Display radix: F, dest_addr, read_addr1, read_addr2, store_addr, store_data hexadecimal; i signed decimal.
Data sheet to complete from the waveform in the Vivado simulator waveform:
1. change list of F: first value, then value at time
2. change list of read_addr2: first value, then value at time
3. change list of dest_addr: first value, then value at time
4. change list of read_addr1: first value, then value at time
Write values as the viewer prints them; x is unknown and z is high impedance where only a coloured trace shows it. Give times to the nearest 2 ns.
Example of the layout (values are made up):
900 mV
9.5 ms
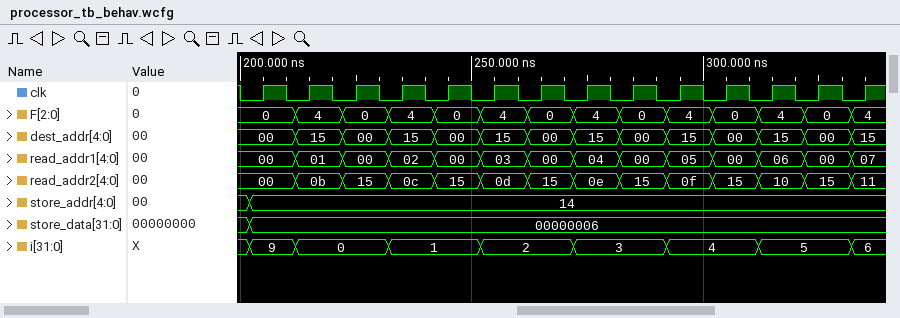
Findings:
0, 4 at 212 ns, 0 at 222 ns, 4 at 232 ns, 0 at 242 ns, 4 at 252 ns, 0 at 262 ns, 4 at 272 ns, 0 at 282 ns, 4 at 292 ns, 0 at 302 ns, 4 at 312 ns, 0 at 322 ns, 4 at 332 ns
00, 0b at 212 ns, 15 at 222 ns, 0c at 232 ns, 15 at 242 ns, 0d at 252 ns, 15 at 262 ns, 0e at 272 ns, 15 at 282 ns, 0f at 292 ns, 15 at 302 ns, 10 at 312 ns, 15 at 322 ns, 11 at 332 ns
00, 15 at 212 ns, 00 at 222 ns, 15 at 232 ns, 00 at 242 ns, 15 at 252 ns, 00 at 262 ns, 15 at 272 ns, 00 at 282 ns, 15 at 292 ns, 00 at 302 ns, 15 at 312 ns, 00 at 322 ns, 15 at 332 ns
00, 01 at 212 ns, 00 at 222 ns, 02 at 232 ns, 00 at 242 ns, 03 at 252 ns, 00 at 262 ns, 04 at 272 ns, 00 at 282 ns, 05 at 292 ns, 00 at 302 ns, 06 at 312 ns, 00 at 322 ns, 07 at 332 ns
